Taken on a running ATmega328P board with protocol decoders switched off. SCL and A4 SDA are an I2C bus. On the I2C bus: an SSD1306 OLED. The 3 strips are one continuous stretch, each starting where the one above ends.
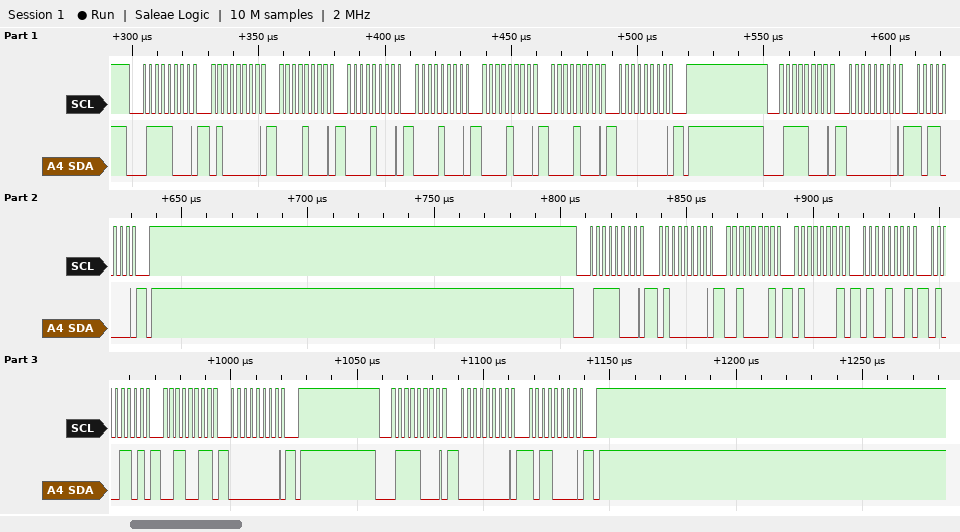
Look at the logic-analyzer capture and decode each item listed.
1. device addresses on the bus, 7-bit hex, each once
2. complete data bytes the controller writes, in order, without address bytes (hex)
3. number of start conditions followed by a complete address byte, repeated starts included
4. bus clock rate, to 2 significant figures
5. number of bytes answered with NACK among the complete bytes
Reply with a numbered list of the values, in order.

1. 0x3C
2. 40 08 08 08 08 08 00 00 B0 40 21 41 49 4D 33 00 00 B0
3. 4
4. 400 kHz
5. 0
